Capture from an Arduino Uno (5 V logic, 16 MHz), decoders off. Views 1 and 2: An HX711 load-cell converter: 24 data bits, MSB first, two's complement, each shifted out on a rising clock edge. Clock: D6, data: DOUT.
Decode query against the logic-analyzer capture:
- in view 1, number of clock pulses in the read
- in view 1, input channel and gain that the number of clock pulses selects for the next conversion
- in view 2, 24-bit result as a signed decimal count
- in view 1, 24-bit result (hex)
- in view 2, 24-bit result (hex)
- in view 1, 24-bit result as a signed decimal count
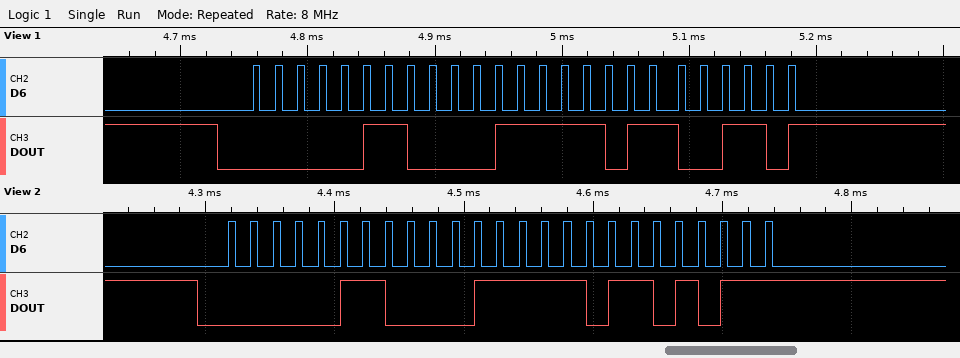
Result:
25
channel A, gain 128
401259
0x061F66
0x061F6B
401254
